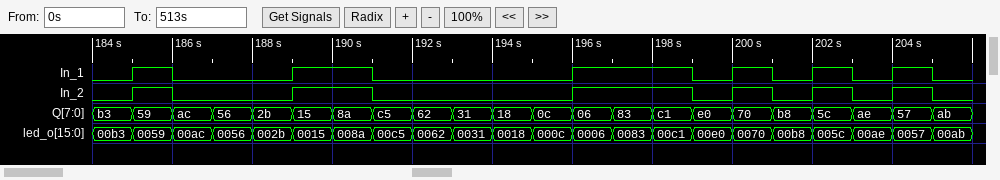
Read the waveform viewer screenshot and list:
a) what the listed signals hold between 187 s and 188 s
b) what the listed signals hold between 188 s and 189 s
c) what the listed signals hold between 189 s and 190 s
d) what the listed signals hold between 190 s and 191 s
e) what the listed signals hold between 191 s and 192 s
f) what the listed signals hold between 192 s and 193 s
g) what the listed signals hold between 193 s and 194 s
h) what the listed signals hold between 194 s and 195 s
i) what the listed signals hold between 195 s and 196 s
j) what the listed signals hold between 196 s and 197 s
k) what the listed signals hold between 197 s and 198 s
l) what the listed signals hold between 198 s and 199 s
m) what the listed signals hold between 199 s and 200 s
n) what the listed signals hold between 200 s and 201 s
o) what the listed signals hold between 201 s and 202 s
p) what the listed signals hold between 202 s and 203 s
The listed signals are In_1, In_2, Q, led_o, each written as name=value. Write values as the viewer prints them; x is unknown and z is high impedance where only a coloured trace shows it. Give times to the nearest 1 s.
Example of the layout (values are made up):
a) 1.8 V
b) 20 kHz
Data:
a) In_1=0, In_2=0, Q=56, led_o=0056
b) In_1=0, In_2=0, Q=2b, led_o=002b
c) In_1=1, In_2=1, Q=15, led_o=0015
d) In_1=1, In_2=1, Q=8a, led_o=008a
e) In_1=0, In_2=0, Q=c5, led_o=00c5
f) In_1=0, In_2=0, Q=62, led_o=0062
g) In_1=0, In_2=0, Q=31, led_o=0031
h) In_1=0, In_2=0, Q=18, led_o=0018
i) In_1=0, In_2=0, Q=0c, led_o=000c
j) In_1=1, In_2=1, Q=06, led_o=0006
k) In_1=1, In_2=1, Q=83, led_o=0083
l) In_1=1, In_2=1, Q=c1, led_o=00c1
m) In_1=0, In_2=0, Q=e0, led_o=00e0
n) In_1=1, In_2=1, Q=70, led_o=0070
o) In_1=0, In_2=0, Q=b8, led_o=00b8
p) In_1=1, In_2=1, Q=5c, led_o=005c
